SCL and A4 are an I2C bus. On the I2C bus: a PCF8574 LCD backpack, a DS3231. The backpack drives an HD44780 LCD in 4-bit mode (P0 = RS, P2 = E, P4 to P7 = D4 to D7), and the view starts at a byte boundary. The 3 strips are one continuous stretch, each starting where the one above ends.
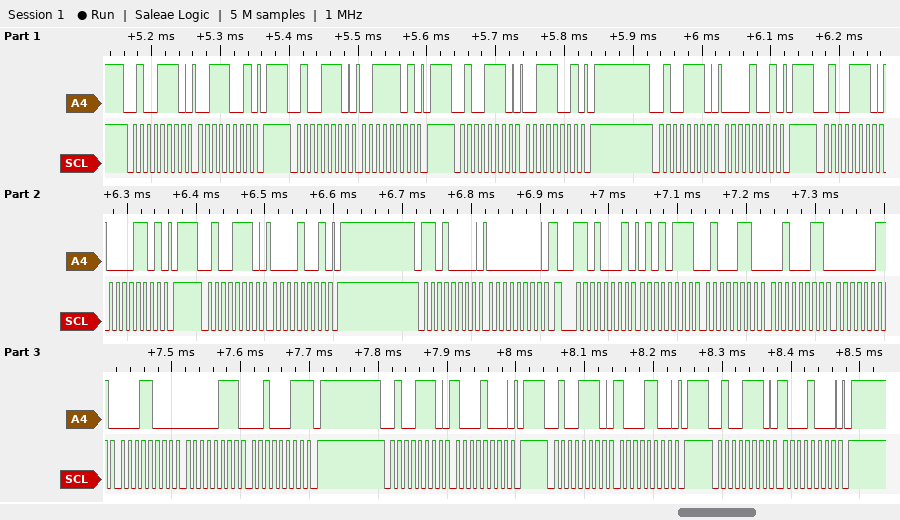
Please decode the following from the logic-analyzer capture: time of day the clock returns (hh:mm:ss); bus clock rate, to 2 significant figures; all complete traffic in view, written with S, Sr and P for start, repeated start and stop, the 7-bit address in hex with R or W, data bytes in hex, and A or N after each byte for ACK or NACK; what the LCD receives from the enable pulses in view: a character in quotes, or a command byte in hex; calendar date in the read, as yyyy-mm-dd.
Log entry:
23:46:57
100 kHz
S 27W A 39 A P S 27W A 3D A P S 27W A 39 A P S 27W A 09 A P S 27W A 0D A P S 27W A 09 A P S 68W A 00 A Sr 68R A 57 A 46 A 23 A 03 A 18 A 07 A 23 N P S 27W A 88 A P S 27W A 8C A P S 27W A 88 A P
'0'
2023-07-18
